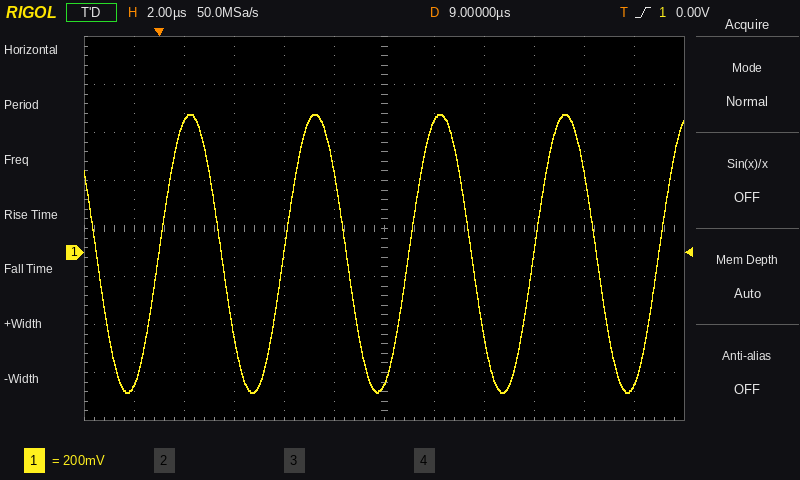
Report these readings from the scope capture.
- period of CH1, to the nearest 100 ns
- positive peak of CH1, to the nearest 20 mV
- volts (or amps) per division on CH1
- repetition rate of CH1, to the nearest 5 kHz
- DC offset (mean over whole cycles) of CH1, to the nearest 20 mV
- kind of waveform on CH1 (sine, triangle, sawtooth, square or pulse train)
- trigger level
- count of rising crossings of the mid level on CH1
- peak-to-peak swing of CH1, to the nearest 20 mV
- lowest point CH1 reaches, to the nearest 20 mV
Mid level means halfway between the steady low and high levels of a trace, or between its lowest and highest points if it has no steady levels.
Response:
5.0 µs
580 mV
200 mV
200 kHz
0 mV
sine
0.00 V
5
1.16 V
-580 mV
